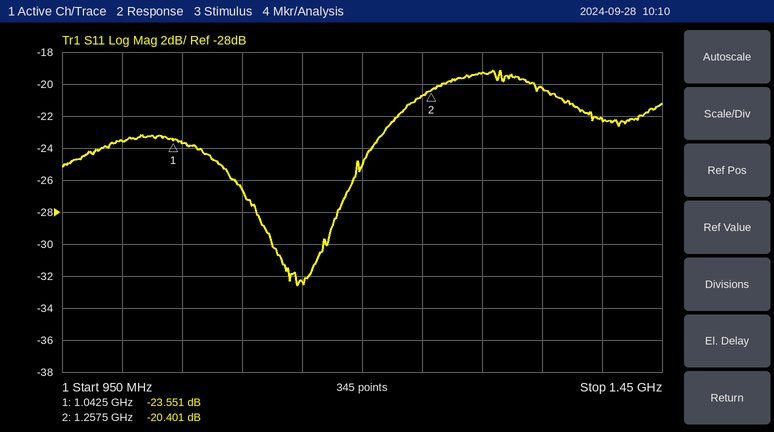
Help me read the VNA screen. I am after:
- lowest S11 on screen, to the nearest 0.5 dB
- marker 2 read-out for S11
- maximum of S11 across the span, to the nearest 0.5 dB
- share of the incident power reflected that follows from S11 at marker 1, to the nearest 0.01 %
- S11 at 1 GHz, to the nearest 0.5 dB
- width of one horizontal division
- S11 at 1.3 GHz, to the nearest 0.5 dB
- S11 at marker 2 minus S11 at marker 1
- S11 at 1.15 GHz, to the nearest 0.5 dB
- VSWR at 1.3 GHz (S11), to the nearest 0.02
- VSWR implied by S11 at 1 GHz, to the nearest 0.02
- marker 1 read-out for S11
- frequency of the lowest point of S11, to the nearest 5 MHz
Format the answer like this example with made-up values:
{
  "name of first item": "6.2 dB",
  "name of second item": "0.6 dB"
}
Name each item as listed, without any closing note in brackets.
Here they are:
{
  "lowest S11 on screen, to the nearest 0.5 dB": "-32.5 dB",
  "marker 2 read-out for S11": "-20.401 dB",
  "maximum of S11 across the span, to the nearest 0.5 dB": "-19.0 dB",
  "share of the incident power reflected that follows from S11 at marker 1, to the nearest 0.01 %": "0.44 %",
  "S11 at 1 GHz, to the nearest 0.5 dB": "-23.5 dB",
  "width of one horizontal division": "50 MHz",
  "S11 at 1.3 GHz, to the nearest 0.5 dB": "-19.5 dB",
  "S11 at marker 2 minus S11 at marker 1": "3.150 dB",
  "S11 at 1.15 GHz, to the nearest 0.5 dB": "-32.5 dB",
  "VSWR at 1.3 GHz (S11), to the nearest 0.02": "1.24",
  "VSWR implied by S11 at 1 GHz, to the nearest 0.02": "1.14",
  "marker 1 read-out for S11": "-23.551 dB",
  "frequency of the lowest point of S11, to the nearest 5 MHz": "1.145 GHz"
}
